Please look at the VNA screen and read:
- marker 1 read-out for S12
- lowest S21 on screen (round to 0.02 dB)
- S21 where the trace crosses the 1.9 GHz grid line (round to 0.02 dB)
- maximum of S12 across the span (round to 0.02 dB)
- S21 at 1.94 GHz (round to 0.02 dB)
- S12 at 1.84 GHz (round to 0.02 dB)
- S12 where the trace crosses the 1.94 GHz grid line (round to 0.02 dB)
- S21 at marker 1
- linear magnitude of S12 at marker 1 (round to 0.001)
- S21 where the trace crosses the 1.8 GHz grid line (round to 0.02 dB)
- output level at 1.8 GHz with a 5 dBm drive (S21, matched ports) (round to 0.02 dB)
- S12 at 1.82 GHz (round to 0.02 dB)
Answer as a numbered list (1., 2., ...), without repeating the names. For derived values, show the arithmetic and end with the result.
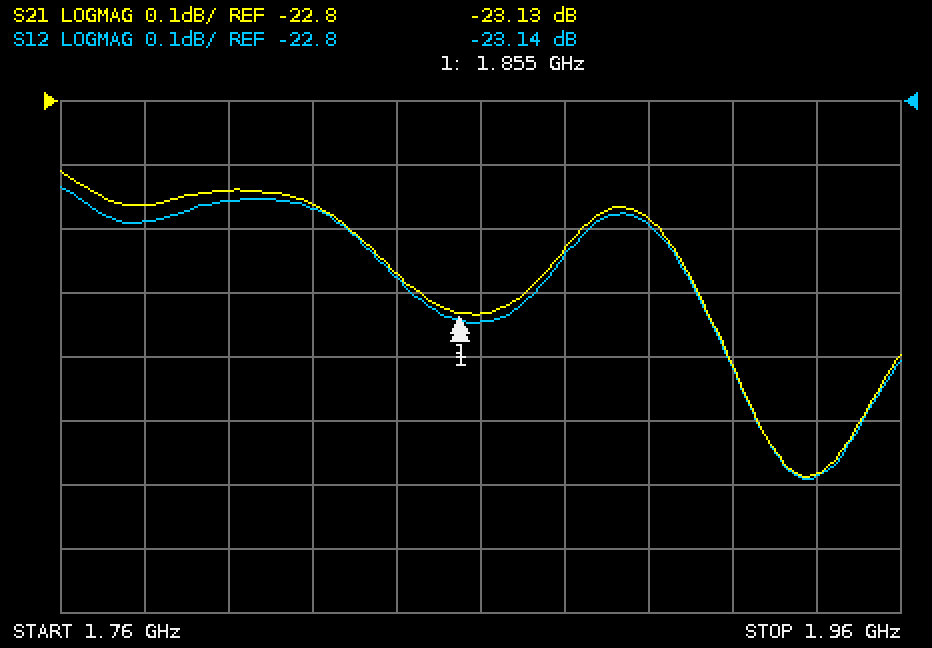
1. -23.14 dB
2. -23.38 dB
3. -22.98 dB
4. -22.94 dB
5. -23.38 dB
6. -23.08 dB
7. -23.38 dB
8. -23.13 dB
9. 10^(-23.14/20) ≈ 0.070
10. -22.94 dB
11. 5 dBm + (-22.94 dB) = -17.94 dBm
12. -22.96 dB
